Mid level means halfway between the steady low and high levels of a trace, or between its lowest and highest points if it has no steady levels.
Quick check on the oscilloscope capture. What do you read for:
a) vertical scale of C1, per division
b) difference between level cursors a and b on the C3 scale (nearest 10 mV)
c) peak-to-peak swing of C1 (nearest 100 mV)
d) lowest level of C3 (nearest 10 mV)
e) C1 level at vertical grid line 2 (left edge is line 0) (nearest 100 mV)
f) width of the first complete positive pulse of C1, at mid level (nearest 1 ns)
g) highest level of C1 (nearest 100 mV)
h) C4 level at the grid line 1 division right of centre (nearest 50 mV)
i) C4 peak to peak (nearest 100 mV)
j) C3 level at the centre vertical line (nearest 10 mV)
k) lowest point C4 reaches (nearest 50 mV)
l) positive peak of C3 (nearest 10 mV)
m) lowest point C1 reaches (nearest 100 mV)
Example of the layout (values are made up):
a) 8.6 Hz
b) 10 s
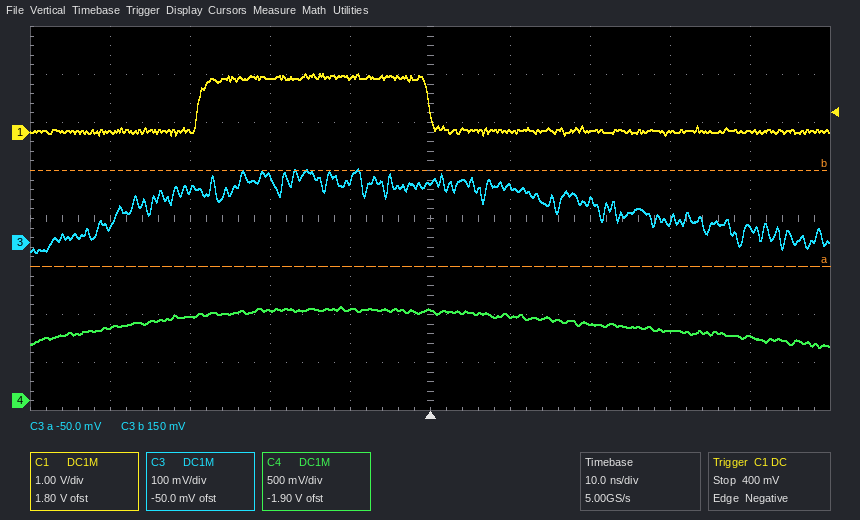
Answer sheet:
a) 1 V
b) 200 mV
c) 1.3 V
d) -20 mV
e) 0.0 V
f) 29 ns
g) 1.2 V
h) 900 mV
i) 400 mV
j) 130 mV
k) 550 mV
l) 150 mV
m) -100 mV
